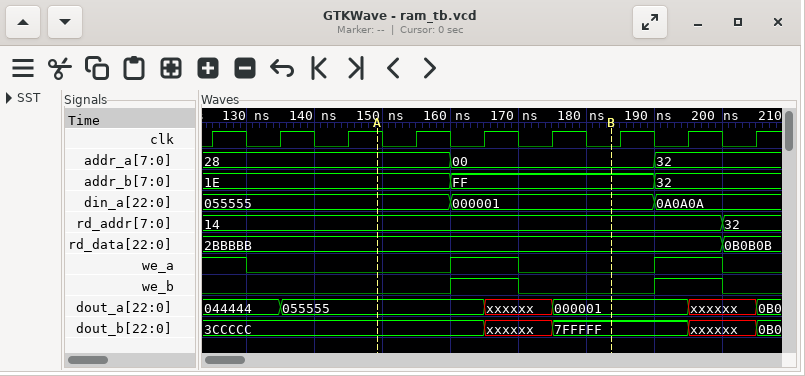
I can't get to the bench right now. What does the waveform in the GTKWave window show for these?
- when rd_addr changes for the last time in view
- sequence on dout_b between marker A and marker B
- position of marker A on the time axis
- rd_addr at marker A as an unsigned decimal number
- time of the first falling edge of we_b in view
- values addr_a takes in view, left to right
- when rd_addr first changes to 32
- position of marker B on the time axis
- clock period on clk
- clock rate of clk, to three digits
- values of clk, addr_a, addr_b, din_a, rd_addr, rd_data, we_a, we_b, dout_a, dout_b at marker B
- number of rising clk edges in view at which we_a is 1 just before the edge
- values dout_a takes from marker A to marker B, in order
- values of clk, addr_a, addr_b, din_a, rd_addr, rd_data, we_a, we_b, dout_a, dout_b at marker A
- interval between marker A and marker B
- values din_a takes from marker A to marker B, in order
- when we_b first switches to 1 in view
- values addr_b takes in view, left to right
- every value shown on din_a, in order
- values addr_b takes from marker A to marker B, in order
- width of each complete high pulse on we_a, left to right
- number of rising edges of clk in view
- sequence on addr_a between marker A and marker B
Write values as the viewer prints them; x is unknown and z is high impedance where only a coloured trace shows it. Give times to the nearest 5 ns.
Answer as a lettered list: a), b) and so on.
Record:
a) 200 ns
b) 3CCCCC, xxxxxx, 7FFFFF
c) 150 ns
d) 20
e) 170 ns
f) 28, 00, 32
g) 200 ns
h) 185 ns
i) 10 ns
j) 100 MHz
k) clk=0, addr_a=00, addr_b=FF, din_a=000001, rd_addr=14, rd_data=2BBBBB, we_a=0, we_b=0, dout_a=000001, dout_b=7FFFFF
l) 3
m) 055555, xxxxxx, 000001
n) clk=1, addr_a=28, addr_b=1E, din_a=055555, rd_addr=14, rd_data=2BBBBB, we_a=0, we_b=0, dout_a=055555, dout_b=3CCCCC
o) 35 ns
p) 055555, 000001
q) 160 ns
r) 1E, FF, 32
s) 055555, 000001, 0A0A0A
t) 1E, FF
u) 10 ns, 10 ns
v) 9
w) 28, 00
